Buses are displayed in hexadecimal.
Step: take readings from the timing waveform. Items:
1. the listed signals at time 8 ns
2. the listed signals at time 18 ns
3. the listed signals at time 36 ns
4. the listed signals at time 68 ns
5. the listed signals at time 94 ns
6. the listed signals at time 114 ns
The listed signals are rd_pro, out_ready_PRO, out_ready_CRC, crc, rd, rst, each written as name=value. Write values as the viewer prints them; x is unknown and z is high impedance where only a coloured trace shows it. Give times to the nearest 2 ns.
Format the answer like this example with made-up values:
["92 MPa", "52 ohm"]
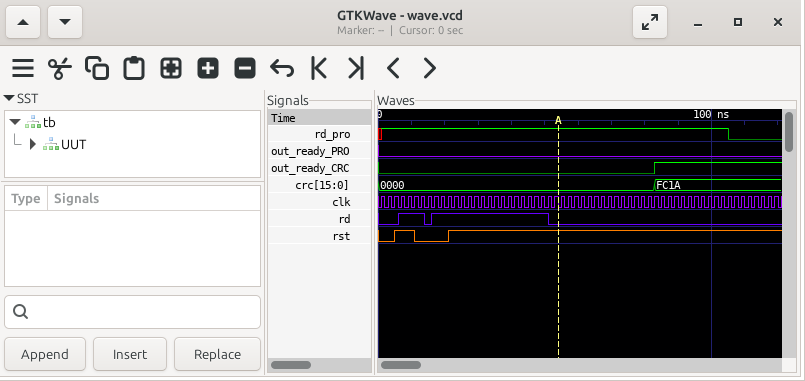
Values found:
["rd_pro=1, out_ready_PRO=0, out_ready_CRC=0, crc=0000, rd=1, rst=1", "rd_pro=1, out_ready_PRO=0, out_ready_CRC=0, crc=0000, rd=1, rst=0", "rd_pro=1, out_ready_PRO=0, out_ready_CRC=0, crc=0000, rd=1, rst=1", "rd_pro=1, out_ready_PRO=0, out_ready_CRC=0, crc=0000, rd=0, rst=1", "rd_pro=1, out_ready_PRO=0, out_ready_CRC=1, crc=FC1A, rd=0, rst=1", "rd_pro=0, out_ready_PRO=0, out_ready_CRC=1, crc=FC1A, rd=0, rst=1"]
